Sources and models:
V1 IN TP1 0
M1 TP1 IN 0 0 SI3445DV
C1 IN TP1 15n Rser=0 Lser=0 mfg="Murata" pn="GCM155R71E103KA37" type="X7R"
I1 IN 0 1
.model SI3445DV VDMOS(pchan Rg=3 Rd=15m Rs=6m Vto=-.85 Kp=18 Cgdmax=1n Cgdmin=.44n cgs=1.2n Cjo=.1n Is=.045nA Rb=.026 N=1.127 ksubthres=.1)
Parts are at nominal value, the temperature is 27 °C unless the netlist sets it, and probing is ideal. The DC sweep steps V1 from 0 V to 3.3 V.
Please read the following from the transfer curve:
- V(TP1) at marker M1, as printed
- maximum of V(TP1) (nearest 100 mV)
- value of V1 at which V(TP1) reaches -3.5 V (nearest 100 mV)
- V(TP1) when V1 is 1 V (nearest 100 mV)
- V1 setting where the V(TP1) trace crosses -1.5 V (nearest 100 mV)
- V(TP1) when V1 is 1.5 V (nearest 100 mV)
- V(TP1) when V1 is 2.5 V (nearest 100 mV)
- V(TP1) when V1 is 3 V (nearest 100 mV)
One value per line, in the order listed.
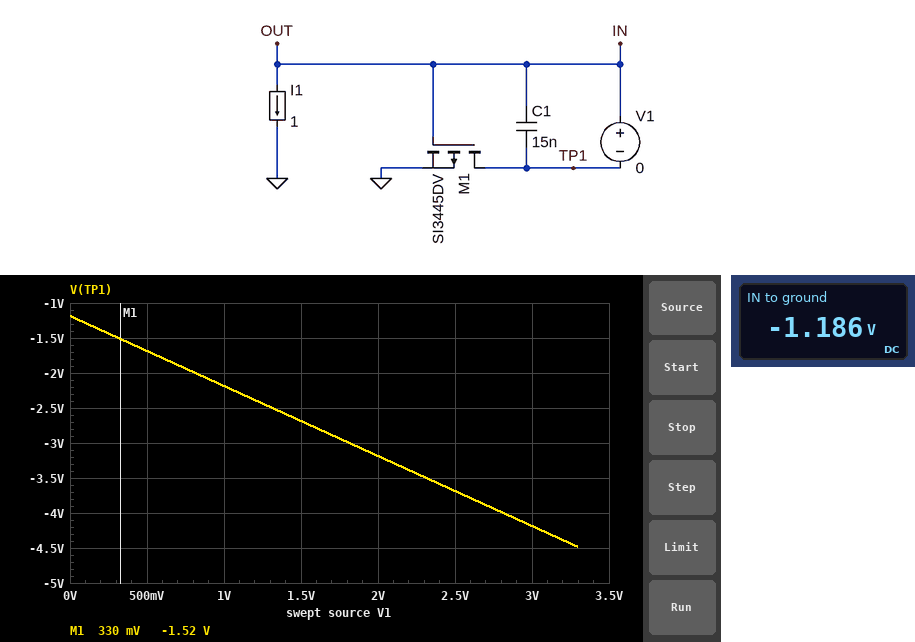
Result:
-1.52 V
-1.2 V
2.3 V
-2.2 V
300 mV
-2.7 V
-3.7 V
-4.2 V
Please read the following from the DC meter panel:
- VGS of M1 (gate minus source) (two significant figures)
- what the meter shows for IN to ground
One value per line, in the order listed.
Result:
-1.2 V
-1.186 V
